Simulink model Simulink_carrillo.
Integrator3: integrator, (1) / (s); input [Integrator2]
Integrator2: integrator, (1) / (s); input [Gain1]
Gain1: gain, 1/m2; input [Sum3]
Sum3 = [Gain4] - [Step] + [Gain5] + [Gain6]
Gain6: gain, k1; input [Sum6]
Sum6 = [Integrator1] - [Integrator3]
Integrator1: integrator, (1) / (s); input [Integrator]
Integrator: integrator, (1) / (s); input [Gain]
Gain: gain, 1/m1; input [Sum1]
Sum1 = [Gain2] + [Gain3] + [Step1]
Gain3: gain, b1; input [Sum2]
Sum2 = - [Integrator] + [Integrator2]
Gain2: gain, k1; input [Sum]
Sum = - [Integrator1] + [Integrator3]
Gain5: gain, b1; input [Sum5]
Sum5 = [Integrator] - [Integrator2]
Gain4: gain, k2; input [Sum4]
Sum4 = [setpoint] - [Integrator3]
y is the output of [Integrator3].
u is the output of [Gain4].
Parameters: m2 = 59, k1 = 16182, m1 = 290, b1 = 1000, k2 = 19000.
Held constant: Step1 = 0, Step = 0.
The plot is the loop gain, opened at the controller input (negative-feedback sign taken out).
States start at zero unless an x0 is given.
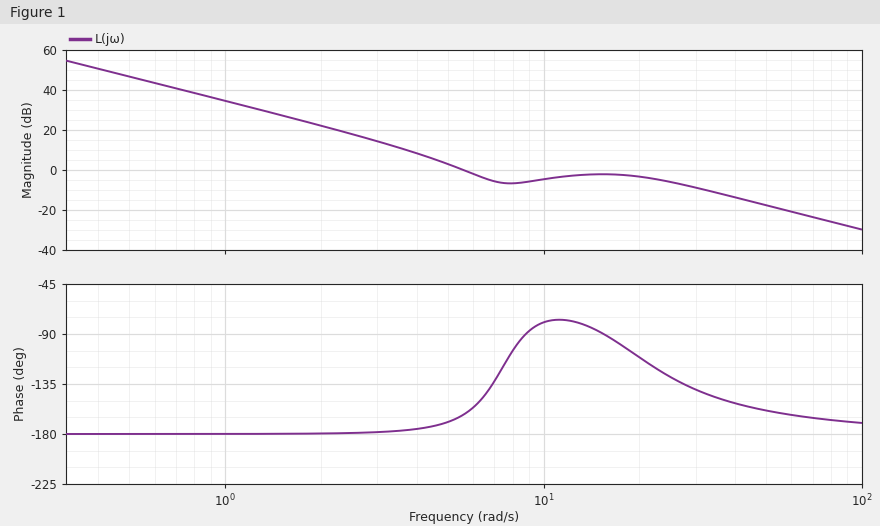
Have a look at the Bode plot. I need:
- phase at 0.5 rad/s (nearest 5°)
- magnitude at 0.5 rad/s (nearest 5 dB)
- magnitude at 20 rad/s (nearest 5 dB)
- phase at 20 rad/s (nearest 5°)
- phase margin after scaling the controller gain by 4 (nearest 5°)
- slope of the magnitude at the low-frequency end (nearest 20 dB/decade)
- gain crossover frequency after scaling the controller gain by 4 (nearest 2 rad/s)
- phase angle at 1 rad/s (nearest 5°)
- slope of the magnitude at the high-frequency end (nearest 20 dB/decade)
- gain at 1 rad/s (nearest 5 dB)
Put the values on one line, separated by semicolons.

-180°; 45 dB; -5 dB; -110°; 30°; -40 dB/decade; 36 rad/s; -180°; -40 dB/decade; 35 dB
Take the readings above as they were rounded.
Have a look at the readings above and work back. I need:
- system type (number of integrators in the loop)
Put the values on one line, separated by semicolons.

2
